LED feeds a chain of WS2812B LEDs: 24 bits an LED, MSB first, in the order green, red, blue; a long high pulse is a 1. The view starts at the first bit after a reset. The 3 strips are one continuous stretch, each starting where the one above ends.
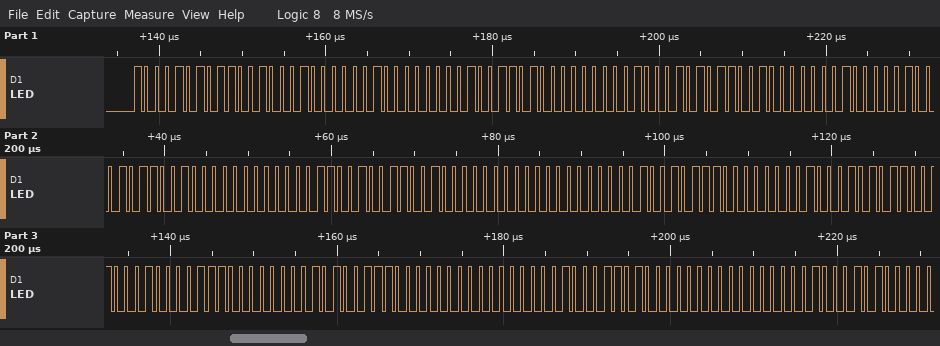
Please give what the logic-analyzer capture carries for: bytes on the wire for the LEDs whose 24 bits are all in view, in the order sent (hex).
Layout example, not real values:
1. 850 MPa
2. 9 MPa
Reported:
1. 8A C8 81 00 9A 00 8A C8 08 22 C8 00 64 C8 00 00 97 00 8A C8 87 00 A7 00 00 8D 00
